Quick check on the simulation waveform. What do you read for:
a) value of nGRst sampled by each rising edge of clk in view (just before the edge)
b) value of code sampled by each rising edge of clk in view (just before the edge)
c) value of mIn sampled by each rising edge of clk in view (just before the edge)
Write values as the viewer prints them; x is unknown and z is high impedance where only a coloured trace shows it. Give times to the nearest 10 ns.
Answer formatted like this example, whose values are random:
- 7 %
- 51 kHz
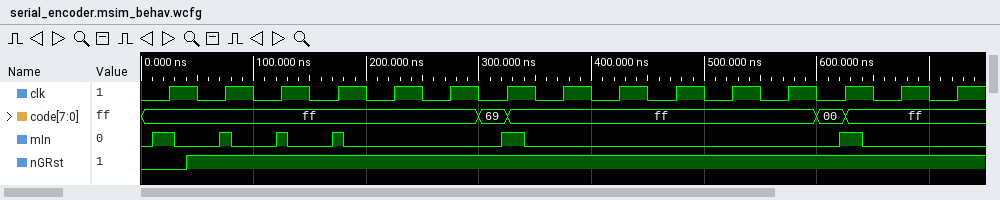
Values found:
- 0 1 1 1 1 1 1 1 1 1 1 1 1 1 1
- ff, ff, ff, ff, ff, ff, 69, ff, ff, ff, ff, ff, 00, ff, ff
- 1 1 1 1 0 0 1 0 0 0 0 0 1 0 0
